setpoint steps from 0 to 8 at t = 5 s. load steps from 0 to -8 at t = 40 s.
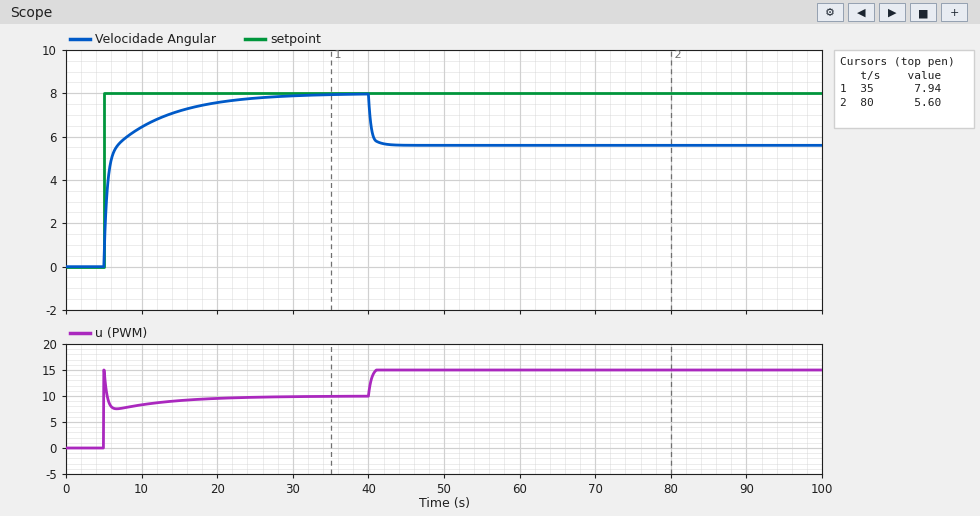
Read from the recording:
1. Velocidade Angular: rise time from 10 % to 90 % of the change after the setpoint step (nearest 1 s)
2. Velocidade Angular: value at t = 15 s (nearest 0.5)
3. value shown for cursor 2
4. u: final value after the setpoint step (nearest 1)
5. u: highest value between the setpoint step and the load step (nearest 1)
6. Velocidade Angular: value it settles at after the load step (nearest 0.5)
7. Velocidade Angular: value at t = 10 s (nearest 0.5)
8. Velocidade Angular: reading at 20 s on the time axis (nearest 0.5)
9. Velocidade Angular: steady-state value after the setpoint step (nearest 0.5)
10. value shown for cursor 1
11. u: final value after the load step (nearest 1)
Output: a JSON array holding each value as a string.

["10 s", "7.0", "5.60", "10", "15", "5.5", "6.5", "7.5", "8.0", "7.94", "15"]
